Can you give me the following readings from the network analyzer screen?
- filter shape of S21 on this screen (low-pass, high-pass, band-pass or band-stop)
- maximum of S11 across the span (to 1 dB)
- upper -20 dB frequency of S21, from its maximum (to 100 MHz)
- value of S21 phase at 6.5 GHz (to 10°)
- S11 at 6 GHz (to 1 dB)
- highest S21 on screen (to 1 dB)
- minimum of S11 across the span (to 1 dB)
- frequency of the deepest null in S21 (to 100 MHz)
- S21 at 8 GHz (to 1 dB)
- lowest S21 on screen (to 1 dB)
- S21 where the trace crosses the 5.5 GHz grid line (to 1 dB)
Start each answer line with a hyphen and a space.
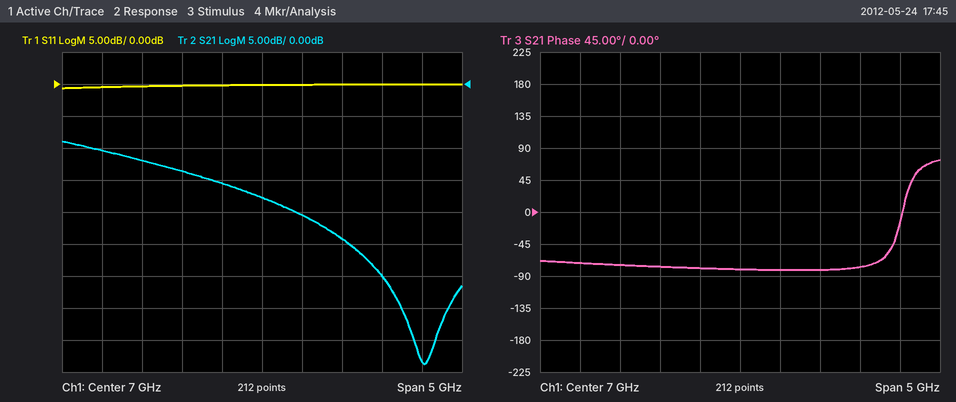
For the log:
- low-pass
- 0 dB
- 8.4 GHz
- -80°
- 0 dB
- -9 dB
- -1 dB
- 9.0 GHz
- -24 dB
- -44 dB
- -12 dB
